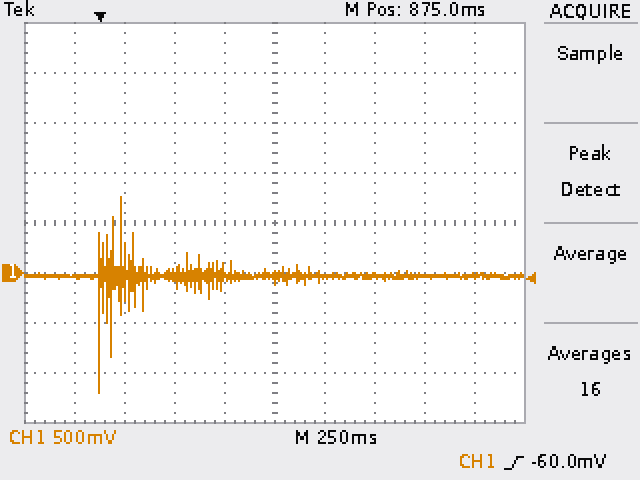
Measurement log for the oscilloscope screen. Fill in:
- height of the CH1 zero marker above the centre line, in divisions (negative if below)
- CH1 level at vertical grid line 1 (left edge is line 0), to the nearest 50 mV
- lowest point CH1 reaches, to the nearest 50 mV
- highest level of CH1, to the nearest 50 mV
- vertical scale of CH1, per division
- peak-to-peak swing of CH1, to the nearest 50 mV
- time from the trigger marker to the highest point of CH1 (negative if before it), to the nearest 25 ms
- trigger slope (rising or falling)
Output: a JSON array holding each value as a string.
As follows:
["-1.0 div", "-50 mV", "-1.20 V", "750 mV", "500 mV", "1.95 V", "+100 ms", "rising"]
